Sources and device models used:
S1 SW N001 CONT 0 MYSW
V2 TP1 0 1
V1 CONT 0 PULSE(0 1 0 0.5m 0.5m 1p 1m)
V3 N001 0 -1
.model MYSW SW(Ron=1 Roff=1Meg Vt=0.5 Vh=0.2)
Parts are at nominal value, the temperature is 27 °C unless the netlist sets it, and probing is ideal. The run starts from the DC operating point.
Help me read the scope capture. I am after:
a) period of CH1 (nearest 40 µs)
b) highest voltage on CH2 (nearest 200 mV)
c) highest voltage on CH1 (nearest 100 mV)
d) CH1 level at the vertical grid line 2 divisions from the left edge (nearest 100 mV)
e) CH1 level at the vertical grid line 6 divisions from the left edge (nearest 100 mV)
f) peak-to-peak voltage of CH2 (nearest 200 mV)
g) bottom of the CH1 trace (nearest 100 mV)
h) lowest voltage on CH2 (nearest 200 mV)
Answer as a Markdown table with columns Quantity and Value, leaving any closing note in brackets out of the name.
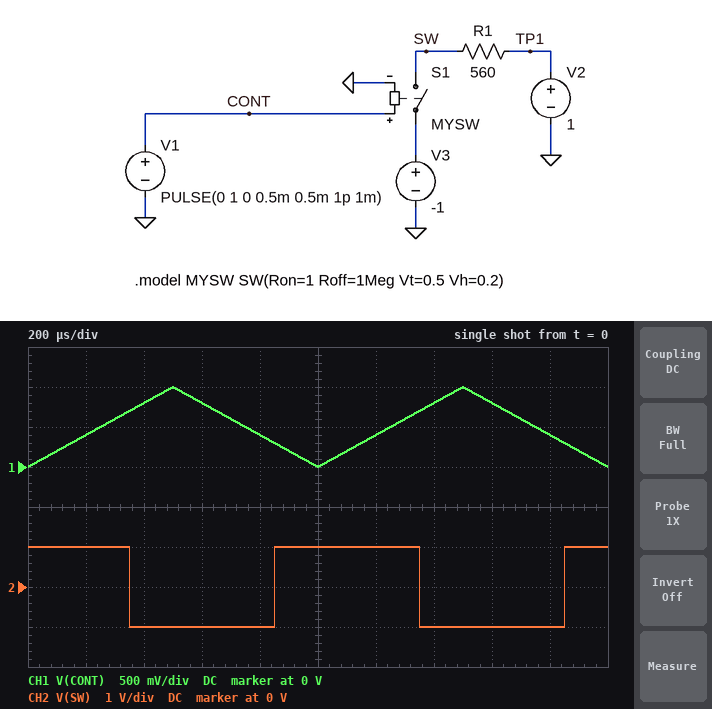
| Quantity | Value |
|---|---|
| period of CH1 | 1.00 ms |
| highest voltage on CH2 | 1.0 V |
| highest voltage on CH1 | 1.0 V |
| CH1 level at the vertical grid line 2 divisions from the left edge | 800 mV |
| CH1 level at the vertical grid line 6 divisions from the left edge | 400 mV |
| peak-to-peak voltage of CH2 | 2.0 V |
| bottom of the CH1 trace | 0 V |
| lowest voltage on CH2 | -1.0 V |
